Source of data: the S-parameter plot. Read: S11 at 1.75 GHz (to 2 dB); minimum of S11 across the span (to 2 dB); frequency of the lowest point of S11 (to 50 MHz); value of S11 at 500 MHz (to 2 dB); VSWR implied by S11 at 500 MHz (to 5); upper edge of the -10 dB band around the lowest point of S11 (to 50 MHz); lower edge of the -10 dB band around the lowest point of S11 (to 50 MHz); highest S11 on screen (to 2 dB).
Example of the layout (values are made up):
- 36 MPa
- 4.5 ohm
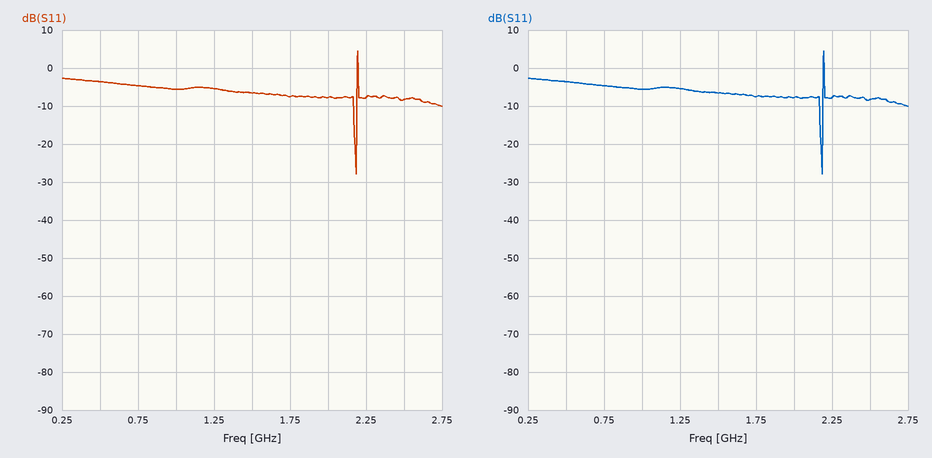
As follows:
- -8 dB
- -28 dB
- 2.20 GHz
- -4 dB
- 5
- 2.20 GHz
- 2.15 GHz
- 4 dB
